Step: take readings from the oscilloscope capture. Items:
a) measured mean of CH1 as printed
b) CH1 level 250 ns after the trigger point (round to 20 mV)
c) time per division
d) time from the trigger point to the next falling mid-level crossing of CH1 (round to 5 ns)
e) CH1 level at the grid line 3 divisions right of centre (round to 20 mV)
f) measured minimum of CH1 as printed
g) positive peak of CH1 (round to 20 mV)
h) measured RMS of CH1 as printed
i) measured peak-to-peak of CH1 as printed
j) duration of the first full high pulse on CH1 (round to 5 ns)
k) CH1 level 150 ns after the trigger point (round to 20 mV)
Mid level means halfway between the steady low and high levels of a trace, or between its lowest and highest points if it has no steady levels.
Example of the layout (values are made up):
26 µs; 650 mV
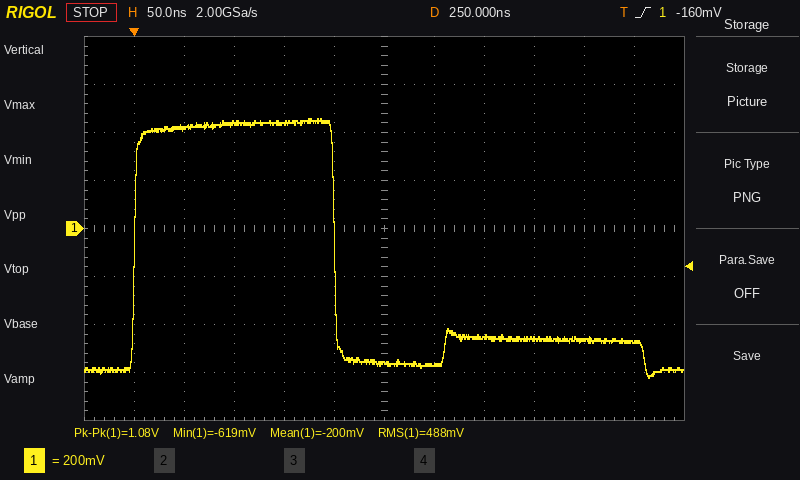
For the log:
-200 mV; -560 mV; 50 ns; 200 ns; -460 mV; -619 mV; 460 mV; 488 mV; 1.08 V; 200 ns; 440 mV
